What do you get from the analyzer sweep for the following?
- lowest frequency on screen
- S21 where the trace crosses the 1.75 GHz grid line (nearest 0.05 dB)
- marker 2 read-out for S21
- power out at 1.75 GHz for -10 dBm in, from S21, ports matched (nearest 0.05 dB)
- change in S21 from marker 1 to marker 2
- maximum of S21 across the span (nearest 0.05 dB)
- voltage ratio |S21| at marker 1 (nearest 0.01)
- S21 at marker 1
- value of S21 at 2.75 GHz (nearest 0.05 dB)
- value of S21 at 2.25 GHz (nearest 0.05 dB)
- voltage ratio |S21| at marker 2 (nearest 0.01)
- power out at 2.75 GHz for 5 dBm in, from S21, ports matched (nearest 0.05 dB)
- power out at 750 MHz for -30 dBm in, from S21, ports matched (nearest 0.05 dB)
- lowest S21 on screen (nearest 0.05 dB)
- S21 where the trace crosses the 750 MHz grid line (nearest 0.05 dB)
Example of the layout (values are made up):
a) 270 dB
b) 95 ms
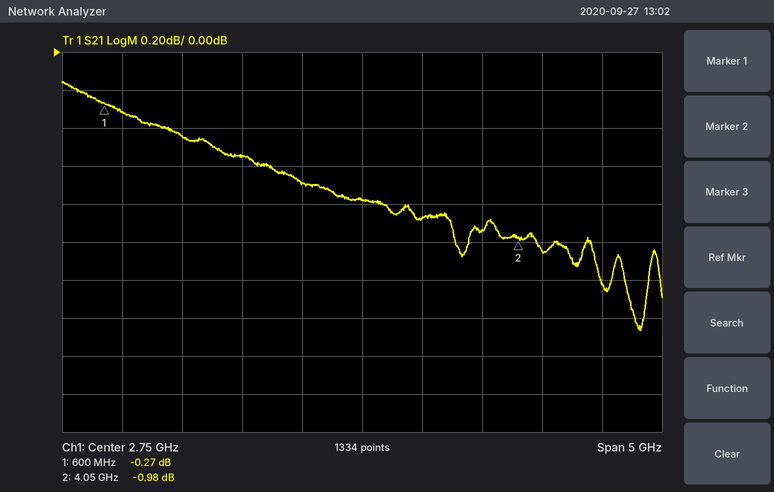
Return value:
a) 250 MHz
b) -0.55 dB
c) -0.98 dB
d) -10.55 dBm
e) -0.71 dB
f) -0.15 dB
g) 0.97
h) -0.27 dB
i) -0.80 dB
j) -0.70 dB
k) 0.89
l) 4.20 dBm
m) -30.30 dBm
n) -1.45 dB
o) -0.30 dB
